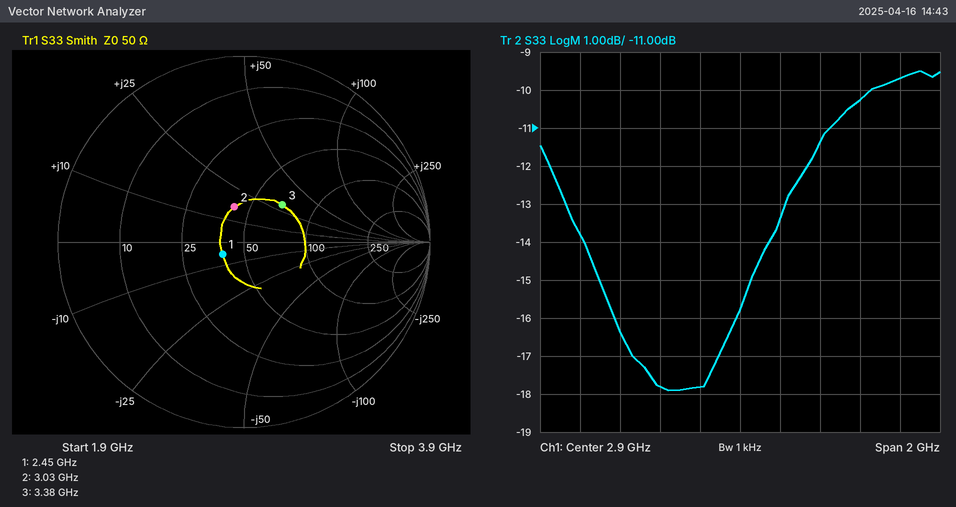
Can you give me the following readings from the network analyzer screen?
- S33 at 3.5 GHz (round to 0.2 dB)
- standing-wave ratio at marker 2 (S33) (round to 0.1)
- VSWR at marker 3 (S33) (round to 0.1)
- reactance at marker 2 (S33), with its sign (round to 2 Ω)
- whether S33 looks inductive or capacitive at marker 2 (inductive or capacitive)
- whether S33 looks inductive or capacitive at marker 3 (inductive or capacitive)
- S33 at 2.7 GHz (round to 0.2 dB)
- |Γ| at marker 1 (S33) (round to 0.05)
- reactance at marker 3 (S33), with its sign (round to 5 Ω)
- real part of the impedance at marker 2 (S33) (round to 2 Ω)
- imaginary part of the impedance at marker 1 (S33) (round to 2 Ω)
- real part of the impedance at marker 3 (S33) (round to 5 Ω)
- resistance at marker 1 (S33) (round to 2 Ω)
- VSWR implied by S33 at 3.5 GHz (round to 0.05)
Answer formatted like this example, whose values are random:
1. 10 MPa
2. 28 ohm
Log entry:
1. -10.2 dB
2. 1.5
3. 1.8
4. +16 Ω
5. inductive
6. inductive
7. -17.8 dB
8. 0.15
9. +30 Ω
10. 42 Ω
11. -6 Ω
12. 70 Ω
13. 40 Ω
14. 1.90
